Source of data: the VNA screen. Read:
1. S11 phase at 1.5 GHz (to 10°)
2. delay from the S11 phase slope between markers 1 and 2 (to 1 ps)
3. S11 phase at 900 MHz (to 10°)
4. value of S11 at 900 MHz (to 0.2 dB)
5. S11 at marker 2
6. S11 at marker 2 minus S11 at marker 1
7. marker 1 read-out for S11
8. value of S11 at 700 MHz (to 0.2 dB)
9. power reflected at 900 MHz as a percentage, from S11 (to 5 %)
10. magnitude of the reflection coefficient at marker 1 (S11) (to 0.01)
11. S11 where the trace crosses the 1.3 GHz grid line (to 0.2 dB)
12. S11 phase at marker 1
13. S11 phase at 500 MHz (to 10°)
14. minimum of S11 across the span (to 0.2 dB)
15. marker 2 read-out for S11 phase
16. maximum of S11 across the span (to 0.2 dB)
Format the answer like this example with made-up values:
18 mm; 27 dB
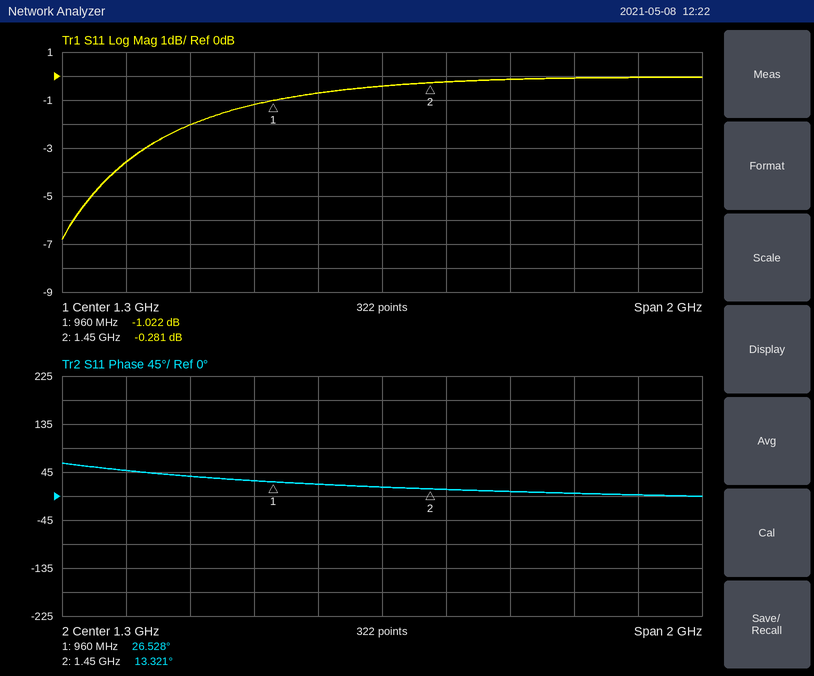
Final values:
10°; 75 ps; 30°; -1.2 dB; -0.281 dB; 0.741 dB; -1.022 dB; -2.0 dB; 75 %; 0.89; -0.4 dB; 26.528°; 50°; -6.8 dB; 13.321°; 0.0 dB
